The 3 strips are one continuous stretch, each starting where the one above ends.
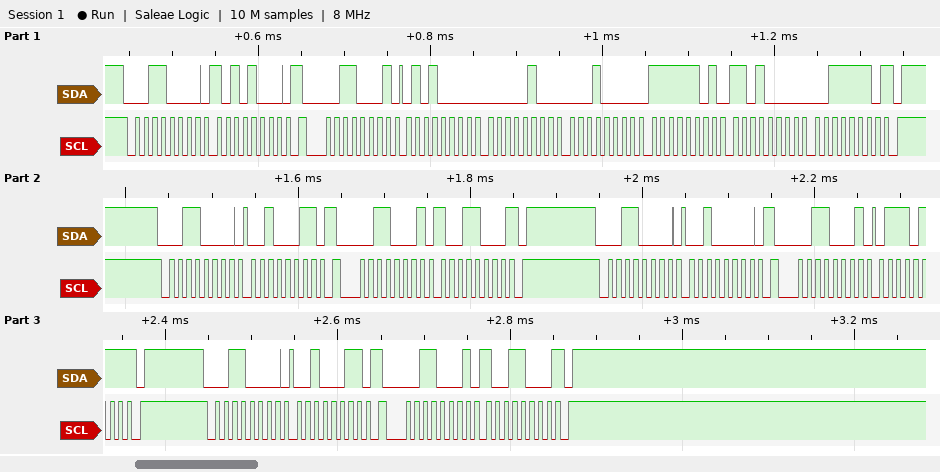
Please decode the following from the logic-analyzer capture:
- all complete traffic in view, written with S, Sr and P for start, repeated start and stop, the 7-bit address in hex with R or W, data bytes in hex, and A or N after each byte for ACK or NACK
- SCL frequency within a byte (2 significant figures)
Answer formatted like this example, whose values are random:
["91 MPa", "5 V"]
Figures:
["S 18W A A8 A Sr 18R A 50 A 04 A 10 A FD A D0 A 3E N P S 18W A 23 A Sr 18R A 98 N P S 18W A 20 A Sr 18R A 77 N P S 18W A 23 A Sr 18R A 98 N P", "100 kHz"]
